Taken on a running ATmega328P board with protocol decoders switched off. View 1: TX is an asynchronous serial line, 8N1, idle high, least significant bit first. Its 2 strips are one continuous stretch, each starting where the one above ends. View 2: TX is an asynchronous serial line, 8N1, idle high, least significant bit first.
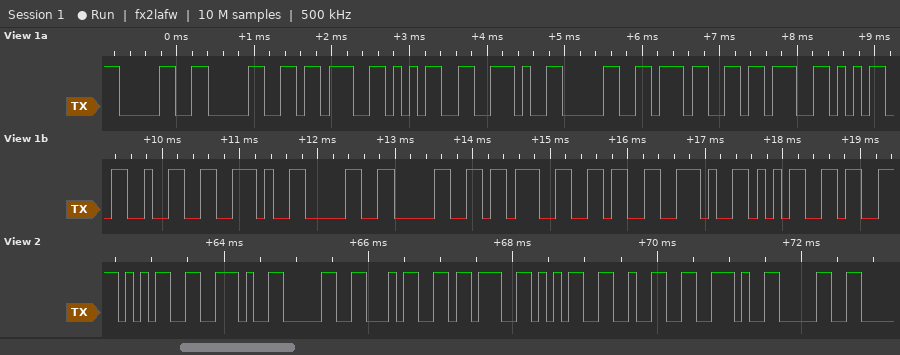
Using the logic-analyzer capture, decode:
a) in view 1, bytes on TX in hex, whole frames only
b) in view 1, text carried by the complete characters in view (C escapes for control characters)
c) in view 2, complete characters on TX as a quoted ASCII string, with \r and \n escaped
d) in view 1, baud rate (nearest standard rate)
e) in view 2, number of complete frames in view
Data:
30 30 3B 35 2E 30 37 3B 35 32 2E 30 30 3B 36 2E 35
"00;5.07;52.00;6.5"
"5.04;52.0"
9600 baud
9
